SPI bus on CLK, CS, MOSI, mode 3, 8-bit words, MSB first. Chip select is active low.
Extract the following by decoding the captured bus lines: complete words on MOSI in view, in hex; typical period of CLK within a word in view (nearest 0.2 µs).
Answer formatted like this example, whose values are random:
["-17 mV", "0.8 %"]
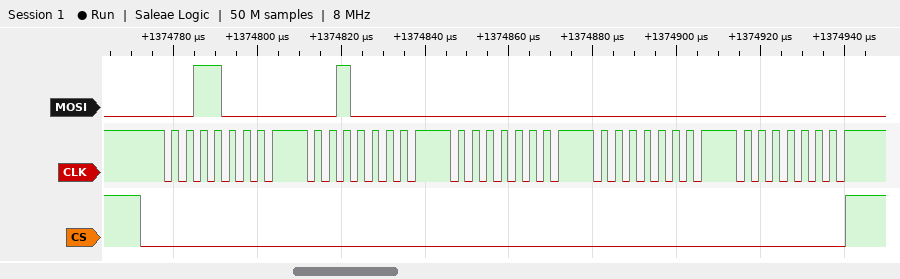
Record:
["30, 20, 00, 00, 00", "3.4 µs"]
